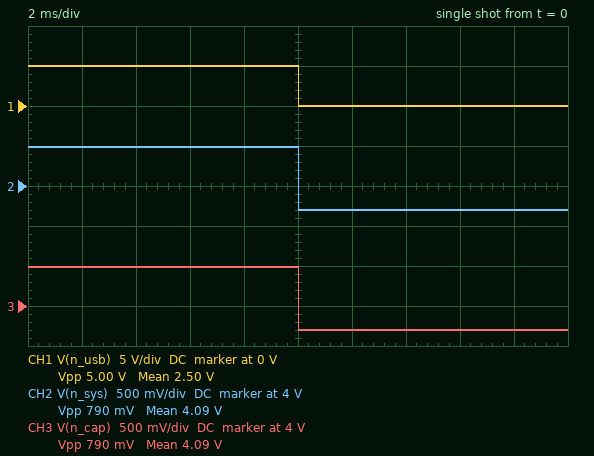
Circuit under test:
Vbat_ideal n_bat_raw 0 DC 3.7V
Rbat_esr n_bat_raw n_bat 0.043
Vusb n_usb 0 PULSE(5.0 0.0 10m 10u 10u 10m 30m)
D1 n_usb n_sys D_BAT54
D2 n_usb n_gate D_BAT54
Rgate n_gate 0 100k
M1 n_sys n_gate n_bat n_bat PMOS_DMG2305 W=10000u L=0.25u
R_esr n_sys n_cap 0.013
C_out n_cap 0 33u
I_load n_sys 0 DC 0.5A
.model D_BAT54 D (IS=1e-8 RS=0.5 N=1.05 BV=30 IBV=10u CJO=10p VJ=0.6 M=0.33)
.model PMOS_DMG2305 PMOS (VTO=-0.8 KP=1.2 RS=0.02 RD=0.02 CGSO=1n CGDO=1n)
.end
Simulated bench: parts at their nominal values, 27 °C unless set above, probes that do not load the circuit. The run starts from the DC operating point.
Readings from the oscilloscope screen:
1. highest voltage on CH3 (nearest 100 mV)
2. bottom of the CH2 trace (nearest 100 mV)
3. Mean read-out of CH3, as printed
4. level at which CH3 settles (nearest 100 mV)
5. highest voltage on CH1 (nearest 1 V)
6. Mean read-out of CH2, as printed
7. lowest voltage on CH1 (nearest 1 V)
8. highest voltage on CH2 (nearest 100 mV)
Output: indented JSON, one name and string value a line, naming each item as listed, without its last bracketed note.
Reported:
{
  "highest voltage on CH3": "4.5 V",
  "bottom of the CH2 trace": "3.7 V",
  "Mean read-out of CH3, as printed": "4.09 V",
  "level at which CH3 settles": "3.7 V",
  "highest voltage on CH1": "5 V",
  "Mean read-out of CH2, as printed": "4.09 V",
  "lowest voltage on CH1": "0 V",
  "highest voltage on CH2": "4.5 V"
}
